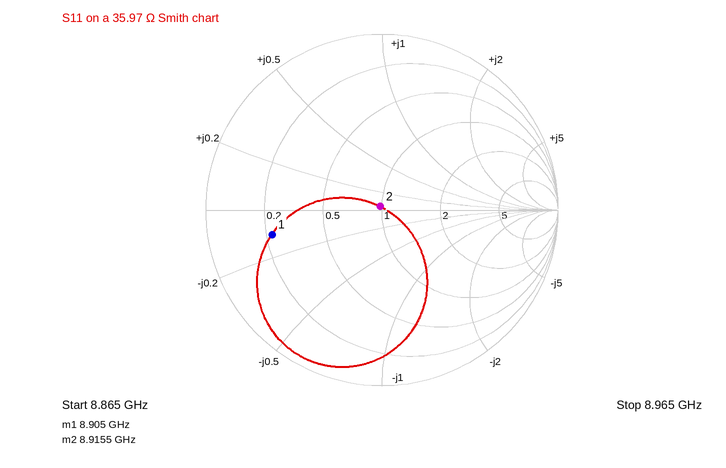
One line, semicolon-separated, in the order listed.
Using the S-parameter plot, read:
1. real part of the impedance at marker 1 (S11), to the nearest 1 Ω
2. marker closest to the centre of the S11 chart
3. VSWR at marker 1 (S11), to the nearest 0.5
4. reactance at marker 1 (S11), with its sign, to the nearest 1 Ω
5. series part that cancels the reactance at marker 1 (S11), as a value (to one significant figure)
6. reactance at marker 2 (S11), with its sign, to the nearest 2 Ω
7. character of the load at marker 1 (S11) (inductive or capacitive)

8 Ω; marker 2; 4.5; -4 Ω; 70 pH; +2 Ω; capacitive
